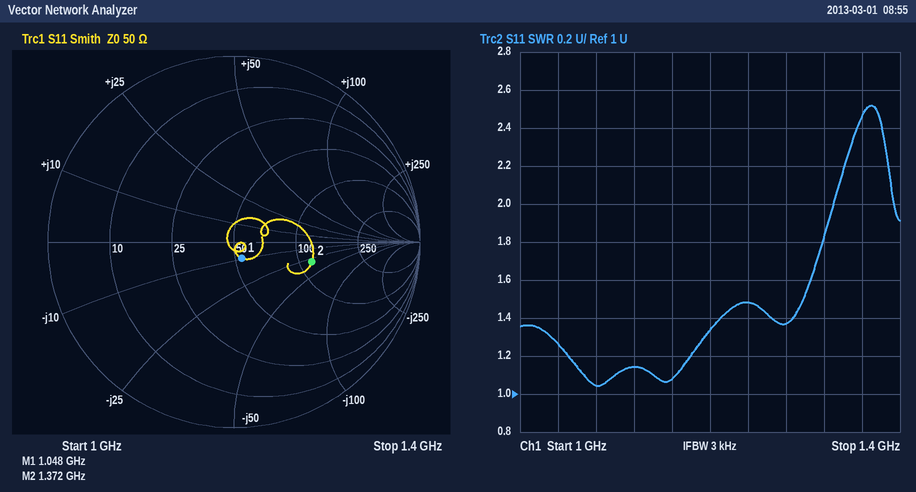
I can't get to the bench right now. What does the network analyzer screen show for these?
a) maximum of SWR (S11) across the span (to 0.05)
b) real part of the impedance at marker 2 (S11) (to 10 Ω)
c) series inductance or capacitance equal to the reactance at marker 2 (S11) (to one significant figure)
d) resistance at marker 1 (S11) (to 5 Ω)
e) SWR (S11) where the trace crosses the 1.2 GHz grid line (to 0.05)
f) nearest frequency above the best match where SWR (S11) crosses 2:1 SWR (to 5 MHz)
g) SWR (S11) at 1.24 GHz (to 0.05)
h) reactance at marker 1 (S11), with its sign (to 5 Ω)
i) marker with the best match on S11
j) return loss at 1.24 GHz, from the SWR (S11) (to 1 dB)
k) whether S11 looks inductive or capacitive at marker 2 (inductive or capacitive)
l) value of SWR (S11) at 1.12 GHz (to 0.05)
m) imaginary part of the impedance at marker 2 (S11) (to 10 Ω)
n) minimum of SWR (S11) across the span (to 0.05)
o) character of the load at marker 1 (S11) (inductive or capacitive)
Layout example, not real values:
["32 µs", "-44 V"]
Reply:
["2.50", "120 Ω", "4 pF", "55 Ω", "1.35", "1.330 GHz", "1.50", "-10 Ω", "marker 1", "14 dB", "capacitive", "1.15", "-30 Ω", "1.05", "capacitive"]
